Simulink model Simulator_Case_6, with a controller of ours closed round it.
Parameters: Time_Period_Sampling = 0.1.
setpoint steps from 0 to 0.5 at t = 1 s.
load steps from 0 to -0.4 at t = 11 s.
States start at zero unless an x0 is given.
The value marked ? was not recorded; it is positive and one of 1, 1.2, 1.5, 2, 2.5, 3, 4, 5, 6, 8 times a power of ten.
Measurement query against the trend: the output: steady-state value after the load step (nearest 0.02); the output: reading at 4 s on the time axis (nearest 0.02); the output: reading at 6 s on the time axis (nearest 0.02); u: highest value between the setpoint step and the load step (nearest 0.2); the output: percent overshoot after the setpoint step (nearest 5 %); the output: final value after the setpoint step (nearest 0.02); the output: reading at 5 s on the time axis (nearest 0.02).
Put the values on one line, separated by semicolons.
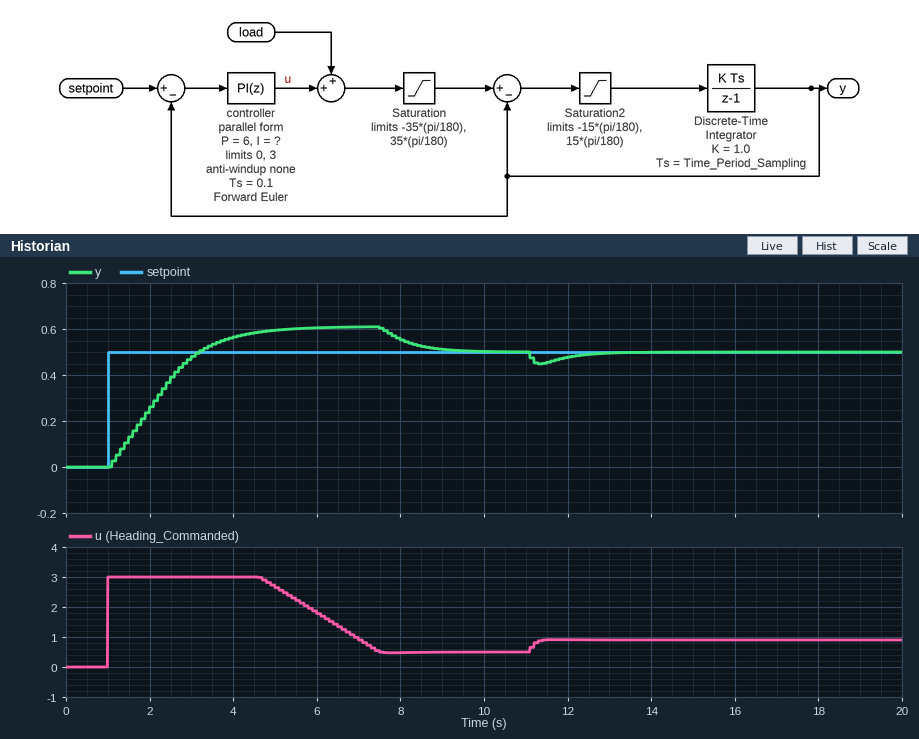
0.50; 0.56; 0.60; 3.0; 20 %; 0.50; 0.60
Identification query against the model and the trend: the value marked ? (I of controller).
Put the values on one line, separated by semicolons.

8
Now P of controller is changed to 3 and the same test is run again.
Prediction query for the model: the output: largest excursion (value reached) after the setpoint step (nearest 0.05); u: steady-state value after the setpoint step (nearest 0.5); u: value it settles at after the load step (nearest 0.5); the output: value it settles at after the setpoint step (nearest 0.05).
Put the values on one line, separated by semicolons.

0.60; 0.5; 1.0; 0.50
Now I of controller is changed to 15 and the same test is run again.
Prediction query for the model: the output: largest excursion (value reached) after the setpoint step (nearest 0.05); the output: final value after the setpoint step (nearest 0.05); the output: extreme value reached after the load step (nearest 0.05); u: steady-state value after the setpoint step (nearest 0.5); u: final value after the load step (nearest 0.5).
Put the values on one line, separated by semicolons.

0.60; 0.50; 0.45; 0.5; 1.0
